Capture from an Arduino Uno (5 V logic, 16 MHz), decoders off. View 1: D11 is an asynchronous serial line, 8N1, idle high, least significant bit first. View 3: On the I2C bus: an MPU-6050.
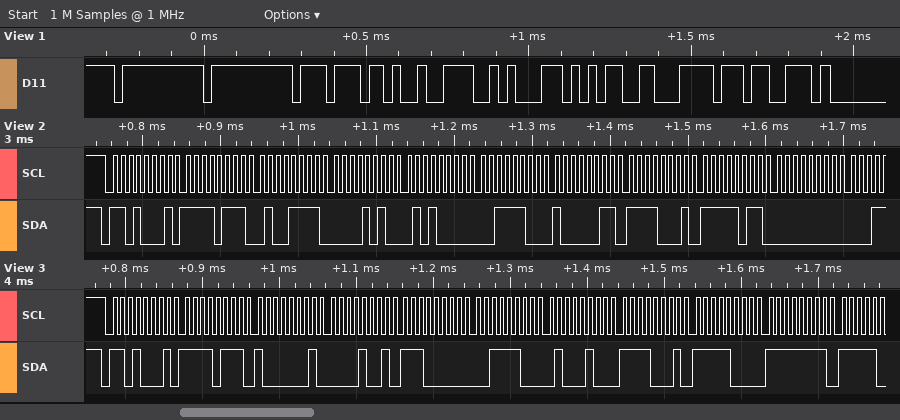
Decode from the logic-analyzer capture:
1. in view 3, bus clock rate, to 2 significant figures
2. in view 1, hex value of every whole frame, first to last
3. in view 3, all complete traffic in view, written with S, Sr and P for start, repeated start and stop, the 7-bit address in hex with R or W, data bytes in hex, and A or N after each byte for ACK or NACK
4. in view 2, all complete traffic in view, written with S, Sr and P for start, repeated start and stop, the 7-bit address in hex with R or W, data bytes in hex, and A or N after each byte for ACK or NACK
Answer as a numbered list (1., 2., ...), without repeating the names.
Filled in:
1. 100 kHz
2. FF FF 77 C9 8A 35 BC 73
3. S 68R A F7 A 81 A 09 A E0 A 3C A 44 A F1 A F8 A FF A
4. S 68R A F7 A 4F A 0A A 50 A 3C A 83 A F1 A FB A 00 A
